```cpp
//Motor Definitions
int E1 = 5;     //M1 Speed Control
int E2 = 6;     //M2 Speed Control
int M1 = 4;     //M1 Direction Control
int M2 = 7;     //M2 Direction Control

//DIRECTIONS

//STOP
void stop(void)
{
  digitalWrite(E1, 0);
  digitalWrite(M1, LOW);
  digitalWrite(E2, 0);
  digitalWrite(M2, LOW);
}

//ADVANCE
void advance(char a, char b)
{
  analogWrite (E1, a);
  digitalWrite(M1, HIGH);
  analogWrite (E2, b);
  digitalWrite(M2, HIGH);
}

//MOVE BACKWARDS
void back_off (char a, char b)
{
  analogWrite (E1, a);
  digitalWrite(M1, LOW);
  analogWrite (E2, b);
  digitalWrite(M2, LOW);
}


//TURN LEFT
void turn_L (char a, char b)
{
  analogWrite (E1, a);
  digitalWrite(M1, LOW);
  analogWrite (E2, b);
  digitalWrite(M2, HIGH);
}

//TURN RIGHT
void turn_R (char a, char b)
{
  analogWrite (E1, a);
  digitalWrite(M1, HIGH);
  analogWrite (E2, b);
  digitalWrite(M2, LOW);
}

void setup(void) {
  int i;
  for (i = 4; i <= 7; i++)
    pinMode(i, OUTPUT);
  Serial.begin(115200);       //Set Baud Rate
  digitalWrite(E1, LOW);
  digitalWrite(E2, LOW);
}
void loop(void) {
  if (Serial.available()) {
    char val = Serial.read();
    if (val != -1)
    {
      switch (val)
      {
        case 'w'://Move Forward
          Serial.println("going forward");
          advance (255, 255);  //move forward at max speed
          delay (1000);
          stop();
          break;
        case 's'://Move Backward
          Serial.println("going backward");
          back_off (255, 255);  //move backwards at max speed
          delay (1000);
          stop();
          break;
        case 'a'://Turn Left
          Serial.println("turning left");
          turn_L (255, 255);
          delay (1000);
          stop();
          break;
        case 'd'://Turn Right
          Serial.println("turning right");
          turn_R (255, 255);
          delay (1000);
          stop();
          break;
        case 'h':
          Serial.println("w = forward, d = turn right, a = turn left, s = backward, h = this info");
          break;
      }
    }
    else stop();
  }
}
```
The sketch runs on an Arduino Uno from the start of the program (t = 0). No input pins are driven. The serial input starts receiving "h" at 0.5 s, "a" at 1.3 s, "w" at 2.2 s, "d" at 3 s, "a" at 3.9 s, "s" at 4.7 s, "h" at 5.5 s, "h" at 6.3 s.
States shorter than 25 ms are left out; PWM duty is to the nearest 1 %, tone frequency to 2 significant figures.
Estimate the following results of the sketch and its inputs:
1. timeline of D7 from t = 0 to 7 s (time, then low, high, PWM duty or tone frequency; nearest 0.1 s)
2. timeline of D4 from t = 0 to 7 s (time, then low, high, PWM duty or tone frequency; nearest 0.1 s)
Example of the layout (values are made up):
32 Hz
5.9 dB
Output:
0 s low; 1.3 s high; 3.3 s low; 4.3 s high; 5.3 s low
0 s low; 2.3 s high; 4.3 s low
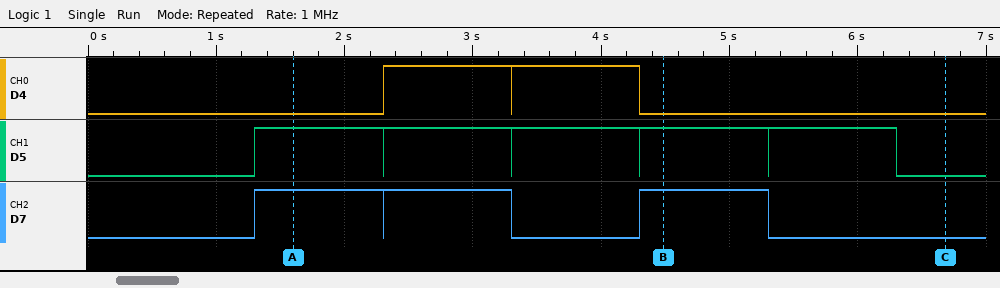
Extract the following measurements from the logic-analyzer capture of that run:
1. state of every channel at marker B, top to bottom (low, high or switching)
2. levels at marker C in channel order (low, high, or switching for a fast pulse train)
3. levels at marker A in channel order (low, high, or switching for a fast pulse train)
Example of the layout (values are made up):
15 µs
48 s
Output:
D4 low, D5 high, D7 high
D4 low, D5 low, D7 low
D4 low, D5 high, D7 high
